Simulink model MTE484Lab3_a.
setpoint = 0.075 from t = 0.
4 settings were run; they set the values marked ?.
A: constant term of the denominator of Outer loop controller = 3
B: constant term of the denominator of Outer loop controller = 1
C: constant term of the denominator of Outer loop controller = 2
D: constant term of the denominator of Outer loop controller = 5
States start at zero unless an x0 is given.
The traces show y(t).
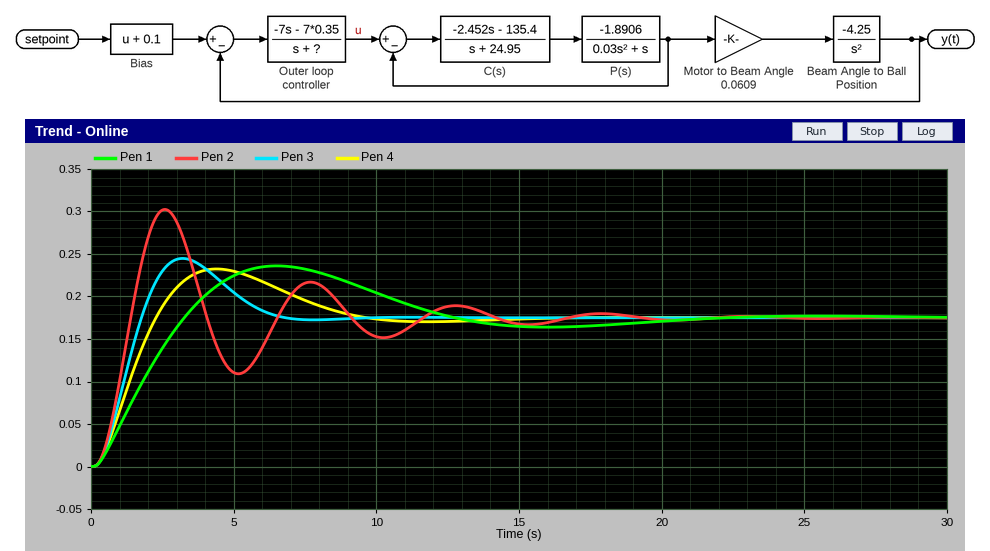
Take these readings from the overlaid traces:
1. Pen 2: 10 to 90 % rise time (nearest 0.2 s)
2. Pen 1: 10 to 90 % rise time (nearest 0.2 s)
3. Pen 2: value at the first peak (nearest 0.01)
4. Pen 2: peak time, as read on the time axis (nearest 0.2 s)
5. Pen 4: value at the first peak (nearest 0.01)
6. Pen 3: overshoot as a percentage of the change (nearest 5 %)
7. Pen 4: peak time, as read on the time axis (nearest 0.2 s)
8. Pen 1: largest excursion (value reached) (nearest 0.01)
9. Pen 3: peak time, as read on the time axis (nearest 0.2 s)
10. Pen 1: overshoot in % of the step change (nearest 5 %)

0.8 s
2.4 s
0.30
2.6 s
0.23
40 %
4.4 s
0.24
3.2 s
35 %
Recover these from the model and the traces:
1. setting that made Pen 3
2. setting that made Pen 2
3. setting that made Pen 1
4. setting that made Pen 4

C
B
D
A
